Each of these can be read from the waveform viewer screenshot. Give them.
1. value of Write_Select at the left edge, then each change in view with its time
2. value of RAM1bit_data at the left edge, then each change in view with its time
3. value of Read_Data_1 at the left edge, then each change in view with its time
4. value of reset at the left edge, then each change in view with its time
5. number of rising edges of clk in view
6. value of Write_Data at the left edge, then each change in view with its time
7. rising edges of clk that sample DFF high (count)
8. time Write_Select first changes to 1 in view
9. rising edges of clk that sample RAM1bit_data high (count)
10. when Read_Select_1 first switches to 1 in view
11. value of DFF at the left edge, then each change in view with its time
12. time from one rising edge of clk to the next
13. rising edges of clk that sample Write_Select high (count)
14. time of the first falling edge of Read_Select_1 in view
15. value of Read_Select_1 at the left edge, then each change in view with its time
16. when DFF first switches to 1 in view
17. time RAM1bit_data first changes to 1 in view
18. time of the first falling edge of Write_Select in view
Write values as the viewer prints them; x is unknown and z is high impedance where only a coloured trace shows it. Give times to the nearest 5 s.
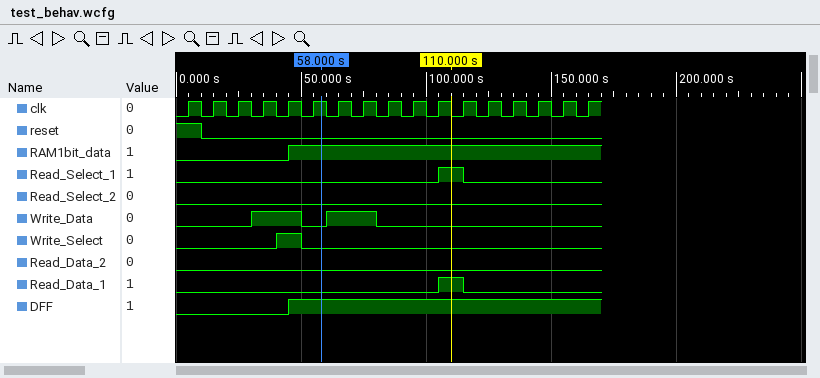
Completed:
0, 1 at 40 s, 0 at 50 s
0, 1 at 45 s
0, 1 at 105 s, 0 at 115 s
1, 0 at 10 s
17
0, 1 at 30 s, 0 at 50 s, 1 at 60 s, 0 at 80 s
12
40 s
12
105 s
0, 1 at 45 s
10 s
1
115 s
0, 1 at 105 s, 0 at 115 s
45 s
45 s
50 s
